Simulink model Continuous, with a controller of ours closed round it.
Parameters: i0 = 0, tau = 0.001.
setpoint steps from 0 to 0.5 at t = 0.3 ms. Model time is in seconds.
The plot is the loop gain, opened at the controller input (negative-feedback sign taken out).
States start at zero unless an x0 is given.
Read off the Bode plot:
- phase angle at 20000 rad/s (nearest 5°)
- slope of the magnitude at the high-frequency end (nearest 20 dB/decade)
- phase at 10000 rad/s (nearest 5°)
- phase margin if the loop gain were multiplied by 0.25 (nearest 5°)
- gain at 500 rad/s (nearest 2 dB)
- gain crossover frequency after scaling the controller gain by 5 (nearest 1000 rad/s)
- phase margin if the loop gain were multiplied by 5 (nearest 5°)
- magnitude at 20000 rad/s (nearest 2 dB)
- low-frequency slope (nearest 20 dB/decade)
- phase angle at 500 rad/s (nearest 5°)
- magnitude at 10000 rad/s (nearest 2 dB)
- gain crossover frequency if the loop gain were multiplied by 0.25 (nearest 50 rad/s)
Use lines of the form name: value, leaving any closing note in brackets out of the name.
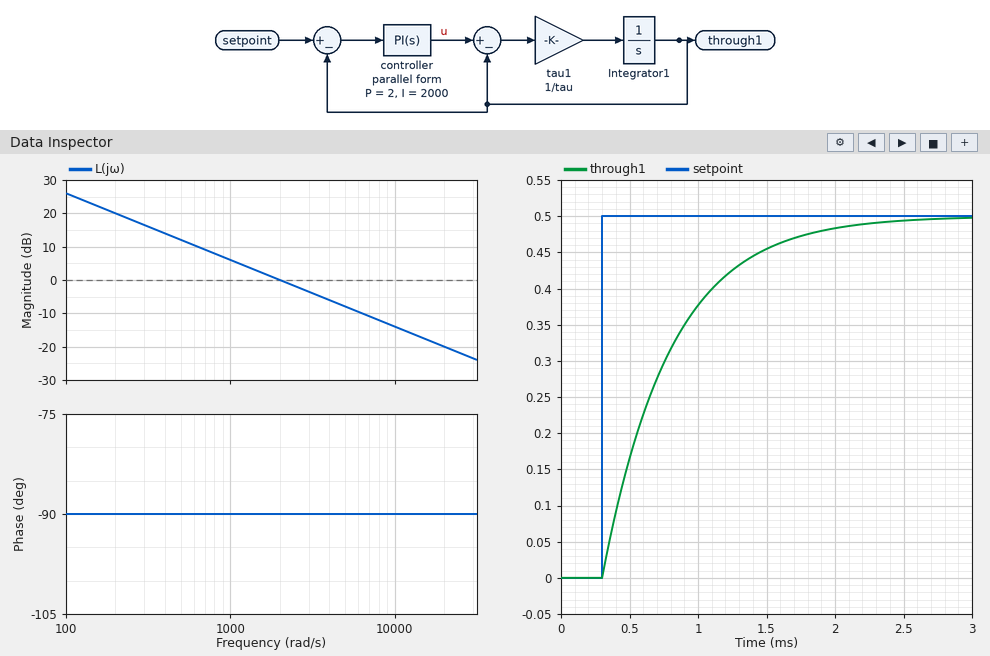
phase angle at 20000 rad/s: -90°
slope of the magnitude at the high-frequency end: -20 dB/decade
phase at 10000 rad/s: -90°
phase margin if the loop gain were multiplied by 0.25: 90°
gain at 500 rad/s: 12 dB
gain crossover frequency after scaling the controller gain by 5: 10000 rad/s
phase margin if the loop gain were multiplied by 5: 90°
magnitude at 20000 rad/s: -20 dB
low-frequency slope: -20 dB/decade
phase angle at 500 rad/s: -90°
magnitude at 10000 rad/s: -14 dB
gain crossover frequency if the loop gain were multiplied by 0.25: 500 rad/s
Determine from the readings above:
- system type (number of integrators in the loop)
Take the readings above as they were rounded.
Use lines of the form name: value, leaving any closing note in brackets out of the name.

system type: 1
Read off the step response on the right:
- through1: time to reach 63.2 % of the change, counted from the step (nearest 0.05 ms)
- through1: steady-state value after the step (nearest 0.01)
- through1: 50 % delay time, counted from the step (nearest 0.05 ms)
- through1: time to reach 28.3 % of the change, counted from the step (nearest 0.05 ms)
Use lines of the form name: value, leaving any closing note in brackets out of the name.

through1: time to reach 63.2 % of the change, counted from the step: 0.50 ms
through1: steady-state value after the step: 0.50
through1: 50 % delay time, counted from the step: 0.35 ms
through1: time to reach 28.3 % of the change, counted from the step: 0.15 ms
